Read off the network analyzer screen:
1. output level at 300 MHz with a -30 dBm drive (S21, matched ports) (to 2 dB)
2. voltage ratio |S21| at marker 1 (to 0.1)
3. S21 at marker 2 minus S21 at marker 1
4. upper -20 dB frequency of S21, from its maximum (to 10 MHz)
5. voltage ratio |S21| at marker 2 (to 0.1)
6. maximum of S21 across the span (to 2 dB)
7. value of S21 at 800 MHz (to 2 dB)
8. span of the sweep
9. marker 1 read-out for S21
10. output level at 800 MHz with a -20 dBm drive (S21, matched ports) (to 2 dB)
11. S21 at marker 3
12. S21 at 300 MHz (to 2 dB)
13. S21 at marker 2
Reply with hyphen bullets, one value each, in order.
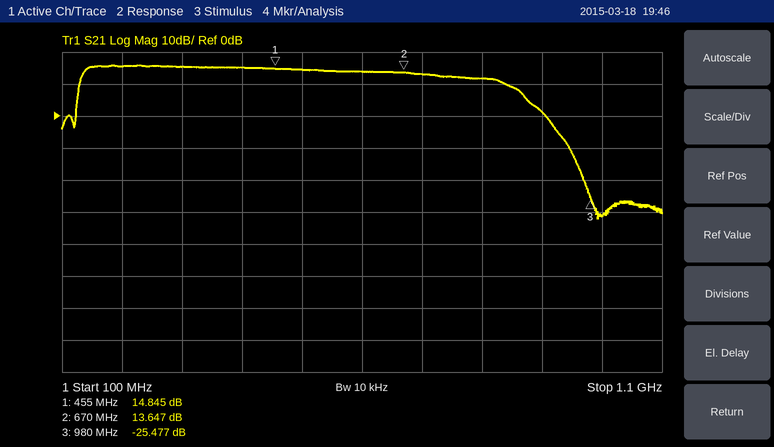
- -14 dBm
- 5.5
- -1.198 dB
- 920 MHz
- 4.8
- 16 dB
- 12 dB
- 1 GHz
- 14.845 dB
- -8 dBm
- -25.477 dB
- 16 dB
- 13.647 dB
